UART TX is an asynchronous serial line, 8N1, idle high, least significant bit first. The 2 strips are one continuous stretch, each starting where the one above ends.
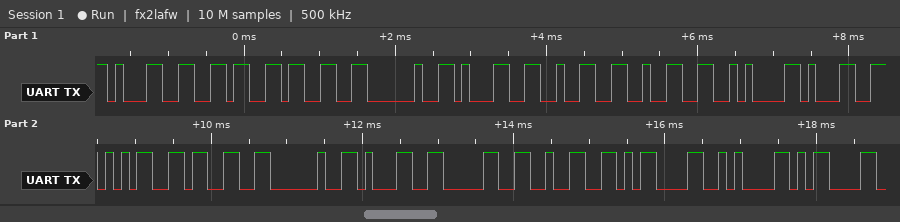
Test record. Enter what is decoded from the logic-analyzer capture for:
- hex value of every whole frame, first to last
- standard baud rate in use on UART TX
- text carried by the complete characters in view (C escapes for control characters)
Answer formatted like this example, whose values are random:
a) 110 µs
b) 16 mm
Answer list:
a) 31 36 33 20 31 32 32 0A 31 35 33 20 31 30 32 0D 0A 0D
b) 9600 baud
c) "163 122\n153 102\r\n\r"
